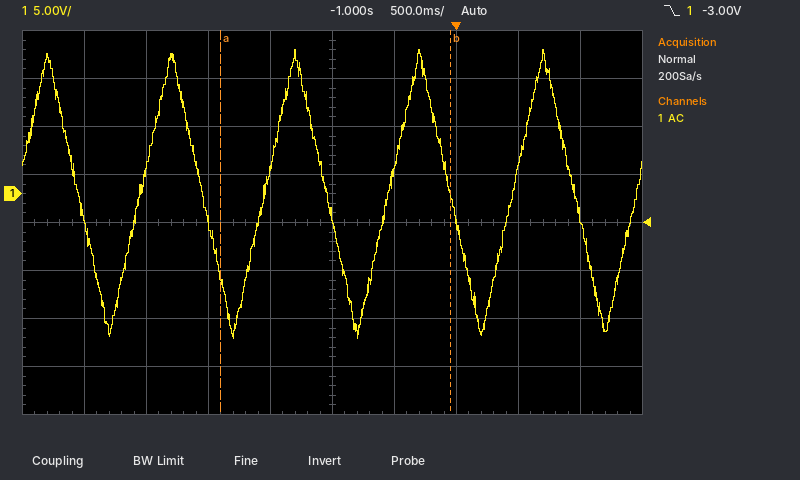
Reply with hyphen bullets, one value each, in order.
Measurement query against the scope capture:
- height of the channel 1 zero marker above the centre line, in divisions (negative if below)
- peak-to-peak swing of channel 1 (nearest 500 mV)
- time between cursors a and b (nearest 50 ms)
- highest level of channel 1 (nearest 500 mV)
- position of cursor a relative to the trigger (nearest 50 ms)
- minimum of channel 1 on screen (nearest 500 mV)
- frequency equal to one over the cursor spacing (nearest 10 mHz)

- +0.6 div
- 30.0 V
- 1.85 s
- 15.0 V
- -1.90 s
- -15.0 V
- 540 mHz
